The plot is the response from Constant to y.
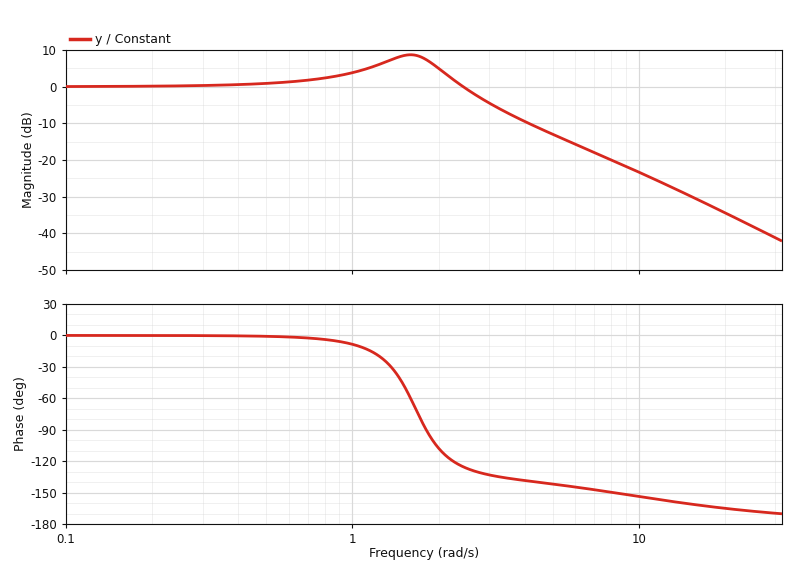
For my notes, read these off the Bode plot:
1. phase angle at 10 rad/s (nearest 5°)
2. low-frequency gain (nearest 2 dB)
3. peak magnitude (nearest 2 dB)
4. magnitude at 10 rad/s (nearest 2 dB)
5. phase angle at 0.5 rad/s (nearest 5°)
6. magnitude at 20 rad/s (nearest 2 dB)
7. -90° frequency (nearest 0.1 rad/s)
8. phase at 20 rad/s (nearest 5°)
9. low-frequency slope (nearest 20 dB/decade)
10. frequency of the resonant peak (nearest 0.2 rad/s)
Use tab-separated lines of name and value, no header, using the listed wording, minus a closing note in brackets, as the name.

phase angle at 10 rad/s	-155°
low-frequency gain	0 dB
peak magnitude	8 dB
magnitude at 10 rad/s	-24 dB
phase angle at 0.5 rad/s	0°
magnitude at 20 rad/s	-34 dB
-90° frequency	1.8 rad/s
phase at 20 rad/s	-165°
low-frequency slope	0 dB/decade
frequency of the resonant peak	1.6 rad/s
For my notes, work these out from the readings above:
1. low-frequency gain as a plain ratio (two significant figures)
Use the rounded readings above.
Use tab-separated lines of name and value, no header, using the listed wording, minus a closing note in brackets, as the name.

low-frequency gain as a plain ratio	1.0
